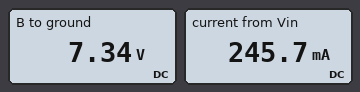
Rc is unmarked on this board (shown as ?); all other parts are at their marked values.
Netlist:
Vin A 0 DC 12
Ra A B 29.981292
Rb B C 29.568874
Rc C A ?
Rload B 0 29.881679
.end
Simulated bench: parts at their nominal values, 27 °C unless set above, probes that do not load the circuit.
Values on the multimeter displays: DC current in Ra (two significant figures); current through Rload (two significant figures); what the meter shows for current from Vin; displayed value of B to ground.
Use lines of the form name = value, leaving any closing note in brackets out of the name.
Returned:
DC current in Ra = 160 mA
current through Rload = 250 mA
what the meter shows for current from Vin = 245.7 mA
displayed value of B to ground = 7.34 V
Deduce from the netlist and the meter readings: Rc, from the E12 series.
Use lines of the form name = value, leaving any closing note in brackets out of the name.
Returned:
Rc, from the E12 series = 22 Ω
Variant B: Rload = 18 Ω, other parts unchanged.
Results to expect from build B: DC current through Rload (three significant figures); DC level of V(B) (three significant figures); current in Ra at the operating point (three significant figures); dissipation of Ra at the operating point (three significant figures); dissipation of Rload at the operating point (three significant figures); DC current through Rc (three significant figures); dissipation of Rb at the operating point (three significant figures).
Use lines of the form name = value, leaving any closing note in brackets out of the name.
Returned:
DC current through Rload = 325 mA
DC level of V(B) = 5.84 V
current in Ra at the operating point = 205 mA
dissipation of Ra at the operating point = 1.26 W
dissipation of Rload at the operating point = 1.90 W
DC current through Rc = 119 mA
dissipation of Rb at the operating point = 421 mW
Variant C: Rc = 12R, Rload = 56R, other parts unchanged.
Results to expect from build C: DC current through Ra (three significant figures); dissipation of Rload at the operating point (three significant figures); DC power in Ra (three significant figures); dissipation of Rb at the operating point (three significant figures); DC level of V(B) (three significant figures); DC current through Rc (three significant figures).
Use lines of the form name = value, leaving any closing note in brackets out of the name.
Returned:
DC current through Ra = 95.0 mA
dissipation of Rload at the operating point = 1.50 W
DC power in Ra = 270 mW
dissipation of Rb at the operating point = 139 mW
DC level of V(B) = 9.15 V
DC current through Rc = 68.5 mA
